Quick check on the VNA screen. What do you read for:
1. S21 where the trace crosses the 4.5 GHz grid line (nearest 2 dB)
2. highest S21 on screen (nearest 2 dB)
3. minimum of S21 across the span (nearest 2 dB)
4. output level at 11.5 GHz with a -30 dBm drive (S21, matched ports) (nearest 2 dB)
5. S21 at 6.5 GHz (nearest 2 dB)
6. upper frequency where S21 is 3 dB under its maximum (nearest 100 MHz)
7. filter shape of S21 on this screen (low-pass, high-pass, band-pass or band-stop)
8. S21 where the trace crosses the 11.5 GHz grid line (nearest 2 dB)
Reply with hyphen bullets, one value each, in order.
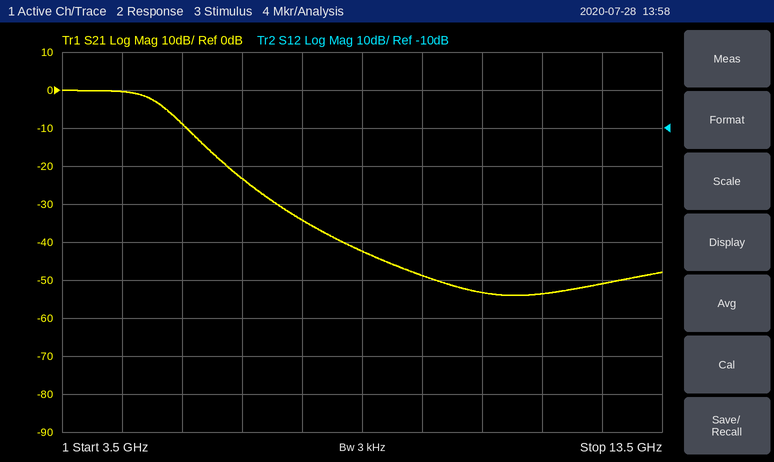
- 0 dB
- 0 dB
- -54 dB
- -84 dBm
- -24 dB
- 5.1 GHz
- low-pass
- -54 dB
